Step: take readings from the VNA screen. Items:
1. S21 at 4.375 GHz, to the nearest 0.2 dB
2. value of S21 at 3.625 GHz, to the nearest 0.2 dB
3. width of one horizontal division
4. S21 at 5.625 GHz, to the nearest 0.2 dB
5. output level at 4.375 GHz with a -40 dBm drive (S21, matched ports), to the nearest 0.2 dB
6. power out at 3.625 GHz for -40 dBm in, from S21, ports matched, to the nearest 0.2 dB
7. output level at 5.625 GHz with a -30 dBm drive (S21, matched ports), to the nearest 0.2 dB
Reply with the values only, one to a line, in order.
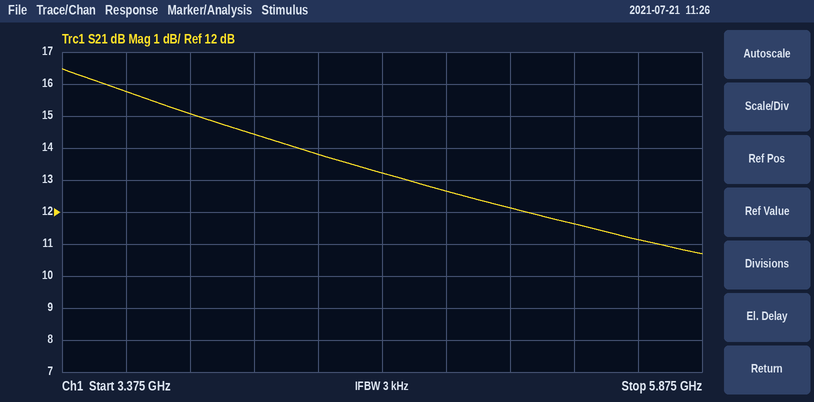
13.8 dB
15.8 dB
250 MHz
11.2 dB
-26.2 dBm
-24.2 dBm
-18.8 dBm
